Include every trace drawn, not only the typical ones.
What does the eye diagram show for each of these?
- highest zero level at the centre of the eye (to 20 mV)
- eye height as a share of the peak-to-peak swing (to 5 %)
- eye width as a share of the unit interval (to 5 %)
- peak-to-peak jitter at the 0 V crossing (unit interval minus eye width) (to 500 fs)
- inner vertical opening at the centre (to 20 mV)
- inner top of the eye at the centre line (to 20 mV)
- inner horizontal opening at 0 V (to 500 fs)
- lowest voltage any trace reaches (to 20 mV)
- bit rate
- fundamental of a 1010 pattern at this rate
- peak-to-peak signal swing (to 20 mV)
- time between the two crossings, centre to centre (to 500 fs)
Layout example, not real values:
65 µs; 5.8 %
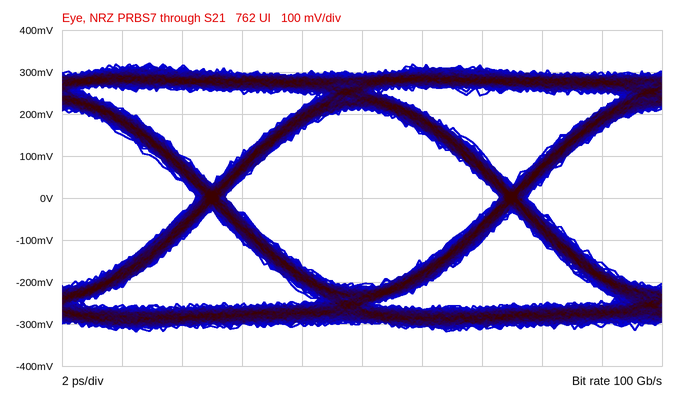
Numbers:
-200 mV; 65 %; 90 %; 1.0 ps; 420 mV; 220 mV; 9.0 ps; -320 mV; 100 Gb/s; 50 GHz; 640 mV; 10.0 ps
